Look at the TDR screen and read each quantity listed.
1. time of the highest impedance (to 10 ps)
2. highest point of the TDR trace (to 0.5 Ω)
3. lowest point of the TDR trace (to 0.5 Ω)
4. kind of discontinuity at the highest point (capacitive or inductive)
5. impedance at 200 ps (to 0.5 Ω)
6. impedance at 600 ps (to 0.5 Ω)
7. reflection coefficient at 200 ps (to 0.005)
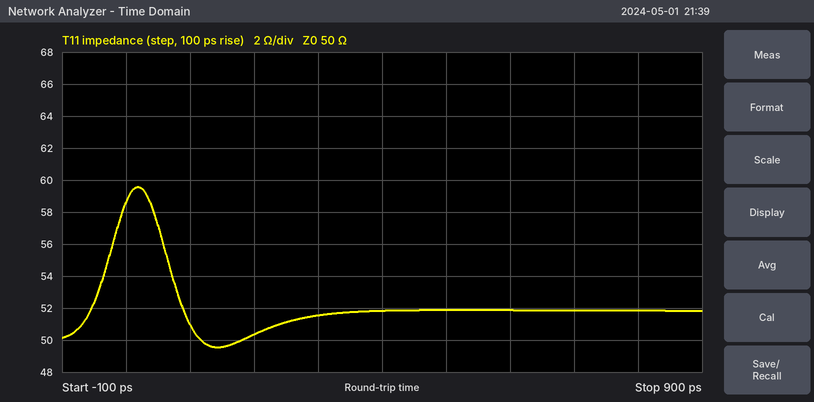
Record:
20 ps
59.5 Ω
49.5 Ω
inductive
50.5 Ω
52.0 Ω
+0.005
